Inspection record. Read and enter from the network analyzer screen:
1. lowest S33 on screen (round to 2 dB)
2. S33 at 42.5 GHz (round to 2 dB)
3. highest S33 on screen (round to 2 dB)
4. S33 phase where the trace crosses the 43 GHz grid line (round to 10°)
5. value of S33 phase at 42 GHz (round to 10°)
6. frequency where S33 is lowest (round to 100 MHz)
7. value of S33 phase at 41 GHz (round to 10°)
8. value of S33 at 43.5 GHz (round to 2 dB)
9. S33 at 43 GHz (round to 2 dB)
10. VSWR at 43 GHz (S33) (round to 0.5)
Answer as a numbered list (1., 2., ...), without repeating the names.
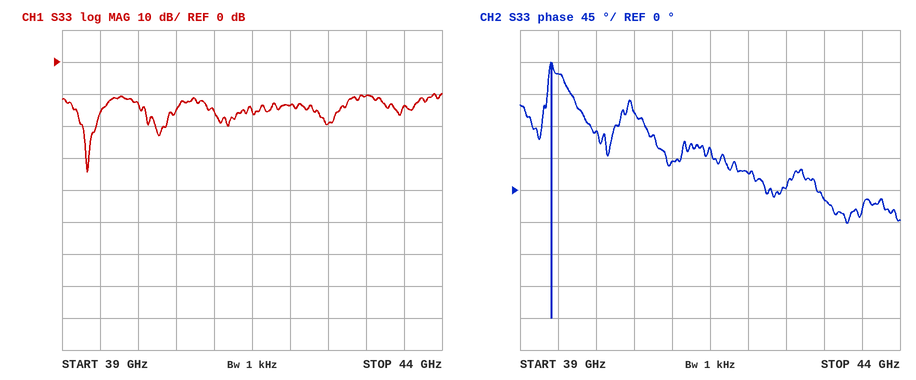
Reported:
1. -34 dB
2. -20 dB
3. -10 dB
4. -10°
5. 20°
6. 39.3 GHz
7. 40°
8. -14 dB
9. -10 dB
10. 2.0
